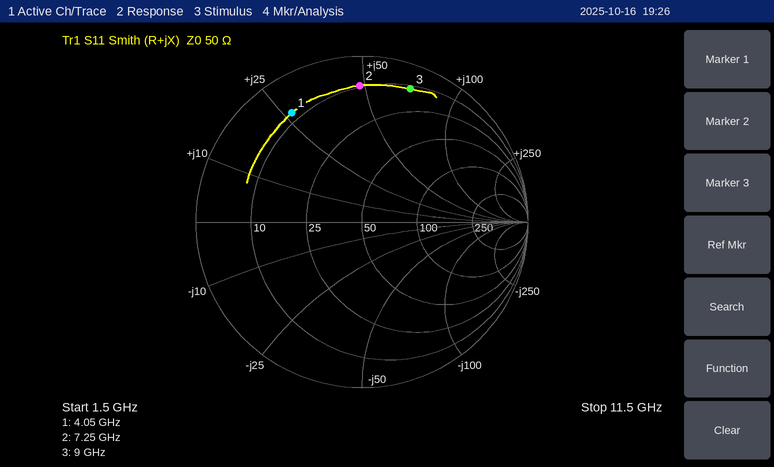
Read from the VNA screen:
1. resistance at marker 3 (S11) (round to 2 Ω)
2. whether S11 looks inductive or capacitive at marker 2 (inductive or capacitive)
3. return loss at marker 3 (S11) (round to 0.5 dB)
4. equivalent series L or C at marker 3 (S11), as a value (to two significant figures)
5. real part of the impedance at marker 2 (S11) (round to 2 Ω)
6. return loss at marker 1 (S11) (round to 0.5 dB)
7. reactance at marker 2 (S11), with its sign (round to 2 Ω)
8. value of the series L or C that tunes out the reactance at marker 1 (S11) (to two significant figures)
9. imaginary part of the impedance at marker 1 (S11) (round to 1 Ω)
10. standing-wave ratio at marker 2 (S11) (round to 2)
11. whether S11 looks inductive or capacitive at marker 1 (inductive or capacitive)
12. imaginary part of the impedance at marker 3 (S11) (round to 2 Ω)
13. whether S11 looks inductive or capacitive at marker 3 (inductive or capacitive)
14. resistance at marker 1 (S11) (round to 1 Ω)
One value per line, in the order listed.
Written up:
12 Ω
inductive
1.5 dB
1.2 nH
10 Ω
2.0 dB
+48 Ω
1.5 pF
+27 Ω
10
inductive
+70 Ω
inductive
8 Ω
